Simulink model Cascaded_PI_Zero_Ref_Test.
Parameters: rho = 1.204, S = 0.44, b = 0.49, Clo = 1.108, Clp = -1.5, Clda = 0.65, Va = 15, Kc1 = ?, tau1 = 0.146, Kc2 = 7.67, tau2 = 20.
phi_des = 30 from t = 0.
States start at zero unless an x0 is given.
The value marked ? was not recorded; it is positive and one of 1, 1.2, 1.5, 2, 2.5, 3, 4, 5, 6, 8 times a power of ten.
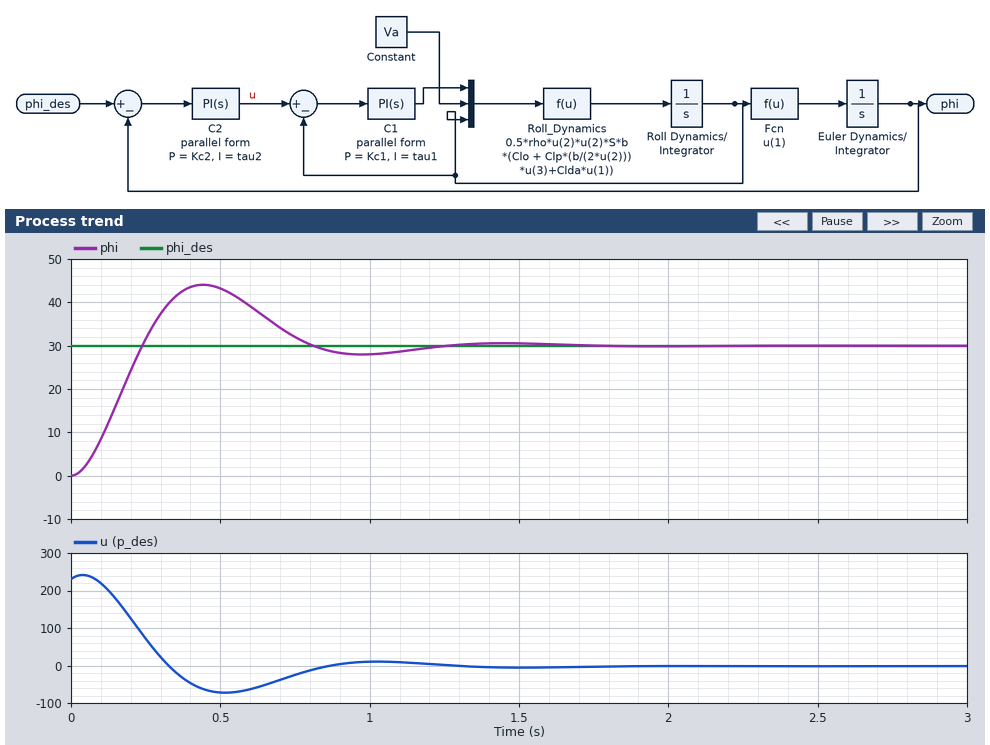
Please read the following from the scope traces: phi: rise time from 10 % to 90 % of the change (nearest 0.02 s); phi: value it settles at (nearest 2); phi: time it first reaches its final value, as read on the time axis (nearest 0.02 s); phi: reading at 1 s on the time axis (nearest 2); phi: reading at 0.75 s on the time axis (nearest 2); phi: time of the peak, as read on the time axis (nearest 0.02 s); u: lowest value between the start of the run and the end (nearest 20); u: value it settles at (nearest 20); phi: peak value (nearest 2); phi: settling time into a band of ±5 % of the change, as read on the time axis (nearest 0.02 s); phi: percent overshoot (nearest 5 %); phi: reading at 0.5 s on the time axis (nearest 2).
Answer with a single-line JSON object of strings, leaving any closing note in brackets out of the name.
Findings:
{"phi: rise time from 10 % to 90 % of the change": "0.16 s", "phi: value it settles at": "30", "phi: time it first reaches its final value, as read on the time axis": "0.24 s", "phi: reading at 1 s on the time axis": "28", "phi: reading at 0.75 s on the time axis": "32", "phi: time of the peak, as read on the time axis": "0.44 s", "u: lowest value between the start of the run and the end": "-80", "u: value it settles at": "0", "phi: peak value": "44", "phi: settling time into a band of ±5 % of the change, as read on the time axis": "1.08 s", "phi: percent overshoot": "45 %", "phi: reading at 0.5 s on the time axis": "44"}
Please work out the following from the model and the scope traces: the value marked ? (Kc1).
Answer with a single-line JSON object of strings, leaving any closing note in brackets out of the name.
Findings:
{"the value marked ?": "0.5"}
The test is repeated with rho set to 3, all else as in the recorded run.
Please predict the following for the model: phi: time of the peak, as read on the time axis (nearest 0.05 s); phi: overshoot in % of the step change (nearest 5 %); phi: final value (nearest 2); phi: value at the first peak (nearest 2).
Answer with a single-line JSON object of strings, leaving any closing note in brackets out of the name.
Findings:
{"phi: time of the peak, as read on the time axis": "0.40 s", "phi: overshoot in % of the step change": "25 %", "phi: final value": "30", "phi: value at the first peak": "38"}
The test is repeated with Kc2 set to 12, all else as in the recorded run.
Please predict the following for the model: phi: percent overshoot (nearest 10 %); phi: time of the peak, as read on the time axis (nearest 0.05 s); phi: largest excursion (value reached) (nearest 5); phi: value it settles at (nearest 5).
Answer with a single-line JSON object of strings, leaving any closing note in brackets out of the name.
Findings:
{"phi: percent overshoot": "40 %", "phi: time of the peak, as read on the time axis": "0.35 s", "phi: largest excursion (value reached)": "40", "phi: value it settles at": "30"}
